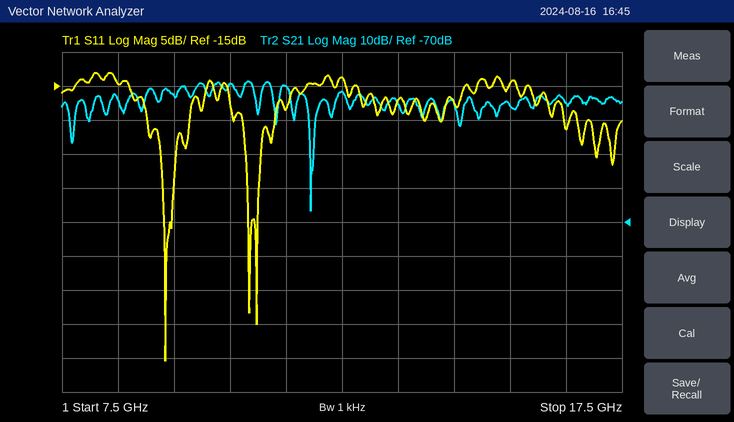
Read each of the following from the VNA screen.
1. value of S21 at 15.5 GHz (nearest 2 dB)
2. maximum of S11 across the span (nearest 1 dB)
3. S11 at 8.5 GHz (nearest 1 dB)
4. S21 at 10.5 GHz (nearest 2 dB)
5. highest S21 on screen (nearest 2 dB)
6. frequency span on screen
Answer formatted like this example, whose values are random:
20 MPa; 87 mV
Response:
-36 dB; -13 dB; -15 dB; -30 dB; -28 dB; 10 GHz
